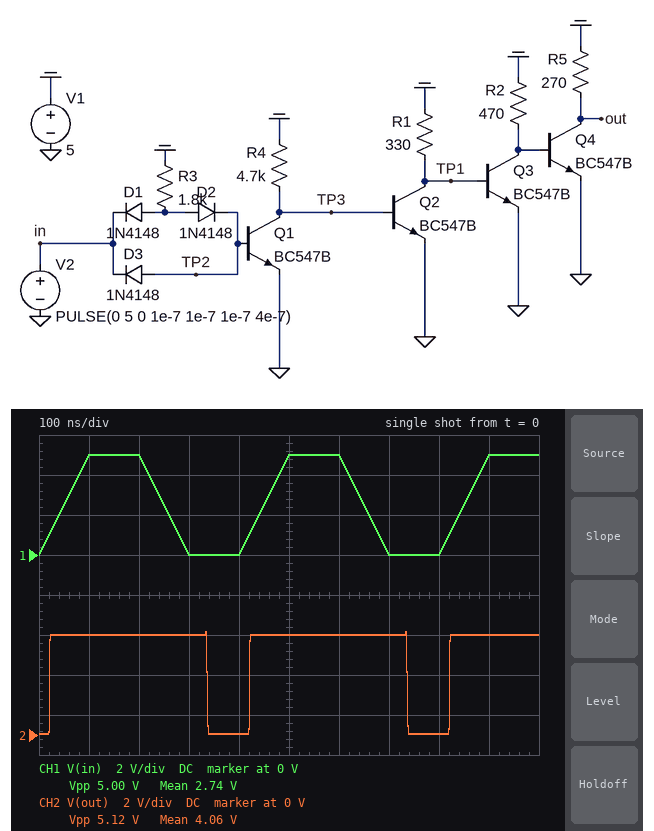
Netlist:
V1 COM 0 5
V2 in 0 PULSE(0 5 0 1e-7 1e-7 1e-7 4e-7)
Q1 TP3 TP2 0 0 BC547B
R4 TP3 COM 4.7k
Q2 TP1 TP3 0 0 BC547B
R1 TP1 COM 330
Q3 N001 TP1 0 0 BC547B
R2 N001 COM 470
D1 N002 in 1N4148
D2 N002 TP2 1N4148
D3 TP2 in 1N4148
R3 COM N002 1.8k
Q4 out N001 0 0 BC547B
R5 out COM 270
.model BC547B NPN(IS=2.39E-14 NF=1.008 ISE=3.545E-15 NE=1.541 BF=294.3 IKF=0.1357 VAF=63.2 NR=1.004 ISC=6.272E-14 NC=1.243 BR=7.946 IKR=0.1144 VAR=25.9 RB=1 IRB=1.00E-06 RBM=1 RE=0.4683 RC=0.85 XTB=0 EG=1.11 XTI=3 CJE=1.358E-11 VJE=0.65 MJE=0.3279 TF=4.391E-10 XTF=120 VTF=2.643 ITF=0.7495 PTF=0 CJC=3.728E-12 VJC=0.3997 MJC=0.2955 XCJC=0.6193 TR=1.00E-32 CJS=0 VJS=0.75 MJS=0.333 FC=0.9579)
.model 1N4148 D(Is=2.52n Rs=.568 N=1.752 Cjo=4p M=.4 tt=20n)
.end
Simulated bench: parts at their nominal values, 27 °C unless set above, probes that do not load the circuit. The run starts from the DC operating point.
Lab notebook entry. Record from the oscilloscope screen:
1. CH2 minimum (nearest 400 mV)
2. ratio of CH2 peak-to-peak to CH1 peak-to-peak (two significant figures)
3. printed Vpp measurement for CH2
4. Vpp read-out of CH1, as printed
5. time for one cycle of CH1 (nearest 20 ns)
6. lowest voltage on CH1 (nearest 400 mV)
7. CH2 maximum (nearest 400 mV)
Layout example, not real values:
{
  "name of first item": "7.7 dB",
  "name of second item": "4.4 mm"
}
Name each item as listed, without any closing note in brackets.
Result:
{
  "CH2 minimum": "0 V",
  "ratio of CH2 peak-to-peak to CH1 peak-to-peak": "1.0",
  "printed Vpp measurement for CH2": "5.12 V",
  "Vpp read-out of CH1, as printed": "5.00 V",
  "time for one cycle of CH1": "400 ns",
  "lowest voltage on CH1": "0 V",
  "CH2 maximum": "5.2 V"
}
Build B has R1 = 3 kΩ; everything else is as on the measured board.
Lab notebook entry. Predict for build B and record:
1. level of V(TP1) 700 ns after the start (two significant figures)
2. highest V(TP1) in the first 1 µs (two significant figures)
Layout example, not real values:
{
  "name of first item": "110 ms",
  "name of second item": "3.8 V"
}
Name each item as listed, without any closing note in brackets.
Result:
{
  "level of V(TP1) 700 ns after the start": "730 mV",
  "highest V(TP1) in the first 1 µs": "740 mV"
}
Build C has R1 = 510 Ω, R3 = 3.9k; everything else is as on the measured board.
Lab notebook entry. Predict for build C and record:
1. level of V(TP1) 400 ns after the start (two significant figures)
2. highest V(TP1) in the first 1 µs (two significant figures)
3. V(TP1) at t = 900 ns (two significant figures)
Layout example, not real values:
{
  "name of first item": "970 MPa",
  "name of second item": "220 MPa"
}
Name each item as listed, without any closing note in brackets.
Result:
{
  "level of V(TP1) 400 ns after the start": "46 mV",
  "highest V(TP1) in the first 1 µs": "780 mV",
  "V(TP1) at t = 900 ns": "770 mV"
}
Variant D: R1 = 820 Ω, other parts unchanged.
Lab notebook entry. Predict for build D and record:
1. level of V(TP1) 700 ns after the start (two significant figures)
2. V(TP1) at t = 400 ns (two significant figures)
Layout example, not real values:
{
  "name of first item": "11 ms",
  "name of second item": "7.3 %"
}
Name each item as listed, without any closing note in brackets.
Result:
{
  "level of V(TP1) 700 ns after the start": "760 mV",
  "V(TP1) at t = 400 ns": "33 mV"
}
